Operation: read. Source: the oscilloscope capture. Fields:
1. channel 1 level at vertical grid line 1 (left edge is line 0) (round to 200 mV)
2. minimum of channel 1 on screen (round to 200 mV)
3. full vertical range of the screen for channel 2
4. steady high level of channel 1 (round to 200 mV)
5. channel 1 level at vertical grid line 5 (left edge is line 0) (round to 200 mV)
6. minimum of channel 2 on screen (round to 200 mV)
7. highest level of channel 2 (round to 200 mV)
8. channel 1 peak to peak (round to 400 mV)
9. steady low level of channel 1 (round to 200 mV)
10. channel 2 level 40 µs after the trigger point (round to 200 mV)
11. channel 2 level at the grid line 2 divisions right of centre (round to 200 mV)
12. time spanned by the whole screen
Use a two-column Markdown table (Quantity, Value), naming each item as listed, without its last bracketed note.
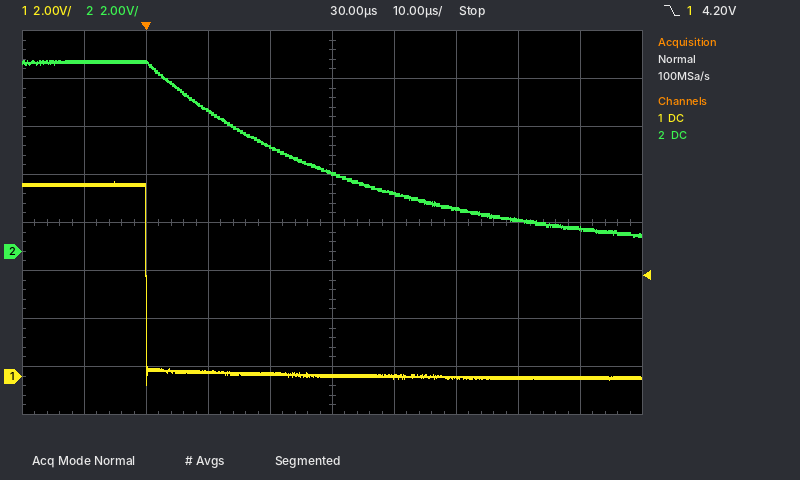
| Quantity | Value |
|---|---|
| channel 1 level at vertical grid line 1 (left edge is line 0) | 8.0 V |
| minimum of channel 1 on screen | -400 mV |
| full vertical range of the screen for channel 2 | 16 V |
| steady high level of channel 1 | 8.0 V |
| channel 1 level at vertical grid line 5 (left edge is line 0) | 0.0 V |
| minimum of channel 2 on screen | 600 mV |
| highest level of channel 2 | 8.0 V |
| channel 1 peak to peak | 8.4 V |
| steady low level of channel 1 | 0.0 V |
| channel 2 level 40 µs after the trigger point | 2.4 V |
| channel 2 level at the grid line 2 divisions right of centre | 1.8 V |
| time spanned by the whole screen | 100 µs |
